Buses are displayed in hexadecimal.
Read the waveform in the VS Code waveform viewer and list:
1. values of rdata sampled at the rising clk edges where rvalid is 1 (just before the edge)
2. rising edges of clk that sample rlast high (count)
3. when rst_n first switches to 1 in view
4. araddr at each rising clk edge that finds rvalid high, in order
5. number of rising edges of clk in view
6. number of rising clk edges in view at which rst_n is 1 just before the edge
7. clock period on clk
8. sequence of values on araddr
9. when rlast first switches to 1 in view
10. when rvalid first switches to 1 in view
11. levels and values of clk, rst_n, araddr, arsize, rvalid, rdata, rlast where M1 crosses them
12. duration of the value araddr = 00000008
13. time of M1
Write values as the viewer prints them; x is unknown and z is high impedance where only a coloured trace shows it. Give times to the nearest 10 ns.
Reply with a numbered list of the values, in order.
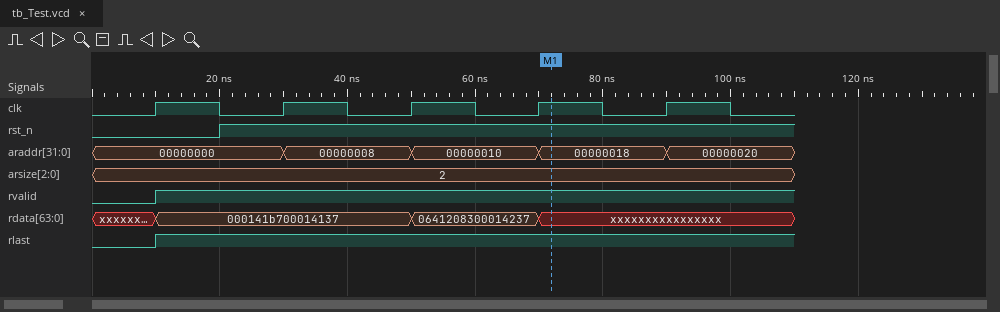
1. 000141b700014137, 000141b700014137, 0641208300014237, xxxxxxxxxxxxxxxx
2. 4
3. 20 ns
4. 00000000, 00000008, 00000010, 00000018
5. 5
6. 4
7. 20 ns
8. 00000000, 00000008, 00000010, 00000018, 00000020
9. 10 ns
10. 10 ns
11. clk=1, rst_n=1, araddr=00000018, arsize=2, rvalid=1, rdata=xxxxxxxxxxxxxxxx, rlast=1
12. 20 ns
13. 70 ns
